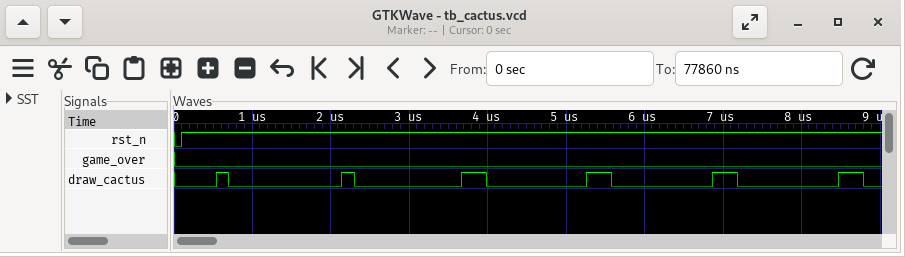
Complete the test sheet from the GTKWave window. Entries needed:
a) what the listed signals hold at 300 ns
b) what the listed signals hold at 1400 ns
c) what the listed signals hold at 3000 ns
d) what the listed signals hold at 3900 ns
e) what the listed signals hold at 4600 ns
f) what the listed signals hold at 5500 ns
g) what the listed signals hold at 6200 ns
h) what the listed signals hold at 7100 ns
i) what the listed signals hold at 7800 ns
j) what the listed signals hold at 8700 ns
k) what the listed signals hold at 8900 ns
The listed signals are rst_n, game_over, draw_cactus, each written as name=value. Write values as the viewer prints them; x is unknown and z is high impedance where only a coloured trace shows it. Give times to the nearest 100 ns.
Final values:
rst_n=1, game_over=0, draw_cactus=0
rst_n=1, game_over=0, draw_cactus=0
rst_n=1, game_over=0, draw_cactus=0
rst_n=1, game_over=0, draw_cactus=1
rst_n=1, game_over=0, draw_cactus=0
rst_n=1, game_over=0, draw_cactus=1
rst_n=1, game_over=0, draw_cactus=0
rst_n=1, game_over=0, draw_cactus=1
rst_n=1, game_over=0, draw_cactus=0
rst_n=1, game_over=0, draw_cactus=1
rst_n=1, game_over=0, draw_cactus=0
